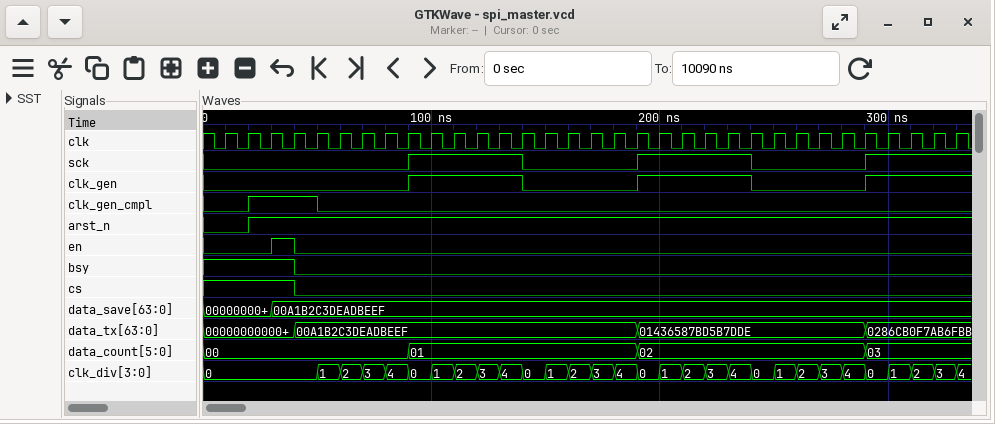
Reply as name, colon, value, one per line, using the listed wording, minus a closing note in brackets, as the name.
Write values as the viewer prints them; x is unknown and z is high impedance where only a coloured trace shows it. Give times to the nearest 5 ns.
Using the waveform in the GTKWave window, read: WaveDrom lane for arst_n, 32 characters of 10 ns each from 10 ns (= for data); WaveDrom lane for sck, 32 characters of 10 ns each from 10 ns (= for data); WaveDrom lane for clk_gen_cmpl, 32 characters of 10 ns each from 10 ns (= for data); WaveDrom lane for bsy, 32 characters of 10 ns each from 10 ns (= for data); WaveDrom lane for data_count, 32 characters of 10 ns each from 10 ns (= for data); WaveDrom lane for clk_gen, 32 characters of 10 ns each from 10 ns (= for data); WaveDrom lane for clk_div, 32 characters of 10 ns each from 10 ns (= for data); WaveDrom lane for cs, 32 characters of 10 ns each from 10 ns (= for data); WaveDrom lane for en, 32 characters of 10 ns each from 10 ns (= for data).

WaveDrom lane for arst_n, 32 characters of 10 ns each from 10 ns: {name: 'arst_n', wave: '01..............................'}
WaveDrom lane for sck, 32 characters of 10 ns each from 10 ns: {name: 'sck', wave: '0.......1....0....1....0....1...'}
WaveDrom lane for clk_gen_cmpl, 32 characters of 10 ns each from 10 ns: {name: 'clk_gen_cmpl', wave: '01..0...........................'}
WaveDrom lane for bsy, 32 characters of 10 ns each from 10 ns: {name: 'bsy', wave: '1..0............................'}
WaveDrom lane for data_count, 32 characters of 10 ns each from 10 ns: {name: 'data_count', wave: '=.......=.........=.........=...', data: '00 01 02 03'}
WaveDrom lane for clk_gen, 32 characters of 10 ns each from 10 ns: {name: 'clk_gen', wave: '0.......1....0....1....0....1...'}
WaveDrom lane for clk_div, 32 characters of 10 ns each from 10 ns: {name: 'clk_div', wave: '=...============================', data: '0 1 2 3 4 0 1 2 3 4 0 1 2 3 4 0 1 2 3 4 0 1 2 3 4 0 1 2 3'}
WaveDrom lane for cs, 32 characters of 10 ns each from 10 ns: {name: 'cs', wave: '1..0............................'}
WaveDrom lane for en, 32 characters of 10 ns each from 10 ns: {name: 'en', wave: '0.10............................'}
